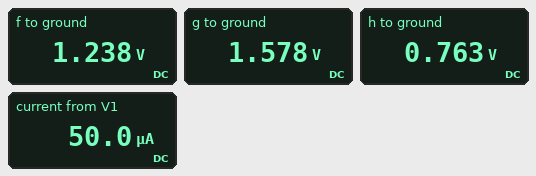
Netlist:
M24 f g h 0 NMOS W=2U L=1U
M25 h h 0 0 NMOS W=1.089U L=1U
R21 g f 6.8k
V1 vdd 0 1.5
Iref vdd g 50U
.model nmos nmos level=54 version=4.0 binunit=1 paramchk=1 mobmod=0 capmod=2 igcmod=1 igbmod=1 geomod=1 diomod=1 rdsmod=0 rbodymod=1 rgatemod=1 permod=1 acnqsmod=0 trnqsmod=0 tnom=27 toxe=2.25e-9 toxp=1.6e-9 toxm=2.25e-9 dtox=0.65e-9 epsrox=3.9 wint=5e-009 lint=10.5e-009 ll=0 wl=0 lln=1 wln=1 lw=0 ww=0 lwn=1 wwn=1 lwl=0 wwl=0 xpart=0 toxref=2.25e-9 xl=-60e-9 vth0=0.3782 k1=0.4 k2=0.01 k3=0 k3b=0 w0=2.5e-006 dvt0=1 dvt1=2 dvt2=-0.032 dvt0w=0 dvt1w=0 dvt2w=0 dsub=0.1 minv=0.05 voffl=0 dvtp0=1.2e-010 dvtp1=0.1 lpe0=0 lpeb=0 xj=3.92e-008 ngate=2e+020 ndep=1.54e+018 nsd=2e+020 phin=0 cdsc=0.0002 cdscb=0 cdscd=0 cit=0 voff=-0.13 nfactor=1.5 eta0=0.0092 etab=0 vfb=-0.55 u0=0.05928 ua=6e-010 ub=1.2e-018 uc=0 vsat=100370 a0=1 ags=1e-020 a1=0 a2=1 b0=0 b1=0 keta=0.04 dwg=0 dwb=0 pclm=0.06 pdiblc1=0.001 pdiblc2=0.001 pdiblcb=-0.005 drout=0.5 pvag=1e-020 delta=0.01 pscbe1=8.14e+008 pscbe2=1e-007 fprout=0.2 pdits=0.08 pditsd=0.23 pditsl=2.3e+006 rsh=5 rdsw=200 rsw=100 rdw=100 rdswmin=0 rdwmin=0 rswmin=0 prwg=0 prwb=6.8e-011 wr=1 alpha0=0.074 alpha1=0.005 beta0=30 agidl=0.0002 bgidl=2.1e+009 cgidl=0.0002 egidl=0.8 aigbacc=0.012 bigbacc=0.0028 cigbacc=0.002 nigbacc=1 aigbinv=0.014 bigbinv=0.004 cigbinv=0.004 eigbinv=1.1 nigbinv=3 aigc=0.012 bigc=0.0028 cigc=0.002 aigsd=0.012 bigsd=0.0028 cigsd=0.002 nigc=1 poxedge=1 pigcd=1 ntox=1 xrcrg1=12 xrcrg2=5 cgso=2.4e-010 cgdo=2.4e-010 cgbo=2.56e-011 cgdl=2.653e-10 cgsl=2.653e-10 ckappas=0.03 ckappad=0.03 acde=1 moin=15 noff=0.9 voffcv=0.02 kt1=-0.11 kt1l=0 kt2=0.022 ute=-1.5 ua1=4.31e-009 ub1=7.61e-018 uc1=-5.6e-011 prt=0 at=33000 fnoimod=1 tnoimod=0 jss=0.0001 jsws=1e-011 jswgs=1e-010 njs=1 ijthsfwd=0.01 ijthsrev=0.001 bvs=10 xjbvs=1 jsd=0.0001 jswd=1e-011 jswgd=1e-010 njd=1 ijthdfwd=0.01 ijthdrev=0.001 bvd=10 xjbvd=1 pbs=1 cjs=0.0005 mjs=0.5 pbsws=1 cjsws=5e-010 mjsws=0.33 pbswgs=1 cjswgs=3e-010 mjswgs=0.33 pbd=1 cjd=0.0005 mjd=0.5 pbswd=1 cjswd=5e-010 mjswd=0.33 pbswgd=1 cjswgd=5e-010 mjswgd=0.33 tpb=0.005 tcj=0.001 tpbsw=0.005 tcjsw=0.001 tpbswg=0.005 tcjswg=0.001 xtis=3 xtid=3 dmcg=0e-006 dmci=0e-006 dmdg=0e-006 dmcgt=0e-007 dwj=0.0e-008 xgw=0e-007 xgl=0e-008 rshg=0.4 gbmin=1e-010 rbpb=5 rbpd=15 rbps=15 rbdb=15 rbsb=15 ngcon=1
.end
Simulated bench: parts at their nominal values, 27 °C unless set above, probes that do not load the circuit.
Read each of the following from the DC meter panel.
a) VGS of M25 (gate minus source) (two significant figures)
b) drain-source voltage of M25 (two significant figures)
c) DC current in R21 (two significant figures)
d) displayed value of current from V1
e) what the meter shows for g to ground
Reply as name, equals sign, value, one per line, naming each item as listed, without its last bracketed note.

VGS of M25 (gate minus source) = 760 mV
drain-source voltage of M25 = 760 mV
DC current in R21 = 50 µA
displayed value of current from V1 = 50.0 µA
what the meter shows for g to ground = 1.578 V
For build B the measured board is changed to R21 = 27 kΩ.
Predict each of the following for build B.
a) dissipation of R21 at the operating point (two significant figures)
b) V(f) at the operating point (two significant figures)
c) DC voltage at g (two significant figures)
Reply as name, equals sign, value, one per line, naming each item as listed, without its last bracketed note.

dissipation of R21 at the operating point = 67 µW
V(f) at the operating point = 830 mV
DC voltage at g = 2.2 V
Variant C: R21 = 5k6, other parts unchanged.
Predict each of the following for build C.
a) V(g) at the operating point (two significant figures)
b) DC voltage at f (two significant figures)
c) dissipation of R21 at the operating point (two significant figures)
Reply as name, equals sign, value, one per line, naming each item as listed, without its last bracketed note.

V(g) at the operating point = 1.6 V
DC voltage at f = 1.3 V
dissipation of R21 at the operating point = 14 µW
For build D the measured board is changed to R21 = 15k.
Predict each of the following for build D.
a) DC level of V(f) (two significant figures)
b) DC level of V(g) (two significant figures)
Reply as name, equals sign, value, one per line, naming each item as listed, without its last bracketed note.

DC level of V(f) = 910 mV
DC level of V(g) = 1.7 V
